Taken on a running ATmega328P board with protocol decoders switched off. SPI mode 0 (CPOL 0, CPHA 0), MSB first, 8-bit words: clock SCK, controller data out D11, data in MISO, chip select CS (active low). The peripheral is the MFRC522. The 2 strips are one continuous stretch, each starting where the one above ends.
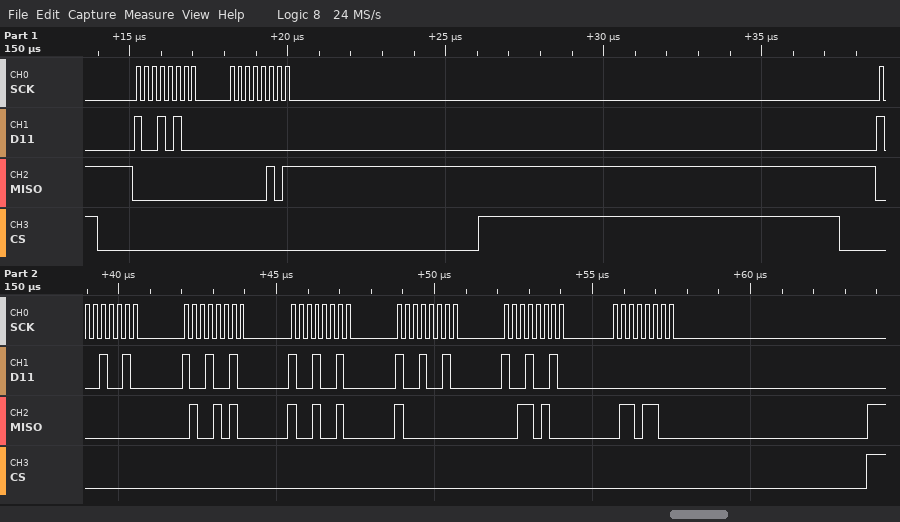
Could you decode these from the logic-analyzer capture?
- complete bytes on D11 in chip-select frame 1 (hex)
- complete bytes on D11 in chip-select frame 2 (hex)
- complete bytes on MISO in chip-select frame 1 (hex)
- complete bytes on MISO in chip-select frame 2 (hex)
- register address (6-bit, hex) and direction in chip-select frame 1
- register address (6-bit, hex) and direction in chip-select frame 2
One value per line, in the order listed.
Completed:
94 00
92 92 92 92 92 00
00 05
00 4A 92 80 34 6C
0x0A read
0x09 read
